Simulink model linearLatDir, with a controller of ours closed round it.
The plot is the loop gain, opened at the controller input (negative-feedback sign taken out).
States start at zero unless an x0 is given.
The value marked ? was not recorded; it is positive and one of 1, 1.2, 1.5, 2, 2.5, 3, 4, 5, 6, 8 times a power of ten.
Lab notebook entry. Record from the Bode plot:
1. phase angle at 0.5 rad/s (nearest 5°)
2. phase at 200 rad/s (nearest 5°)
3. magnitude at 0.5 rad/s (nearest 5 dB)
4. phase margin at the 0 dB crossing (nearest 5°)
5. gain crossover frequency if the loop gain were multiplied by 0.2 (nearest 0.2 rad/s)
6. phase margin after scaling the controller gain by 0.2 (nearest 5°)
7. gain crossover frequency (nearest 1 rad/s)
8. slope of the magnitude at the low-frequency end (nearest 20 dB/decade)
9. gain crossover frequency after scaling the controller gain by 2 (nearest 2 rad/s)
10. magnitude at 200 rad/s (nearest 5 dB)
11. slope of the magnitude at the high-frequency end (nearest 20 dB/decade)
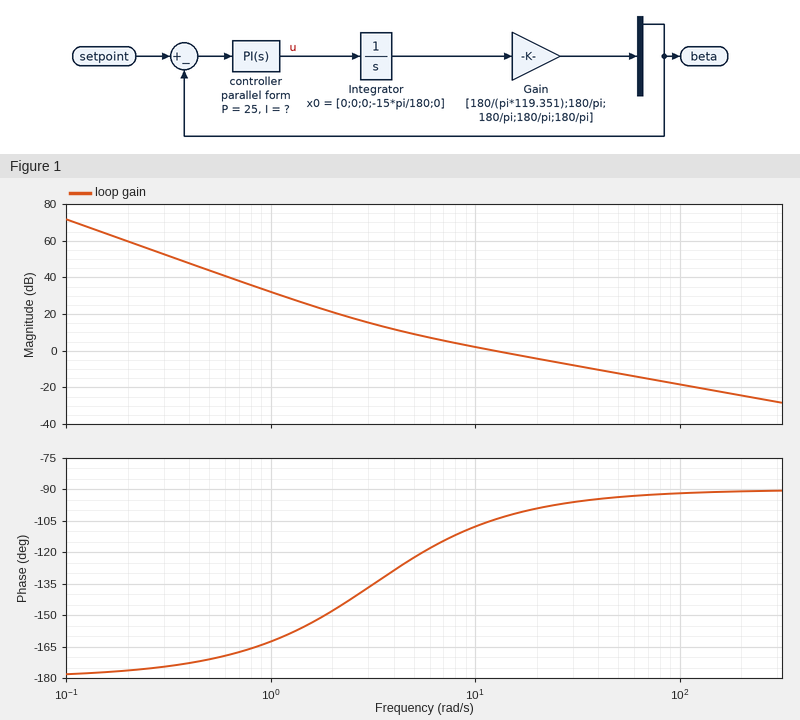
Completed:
-170°
-90°
45 dB
75°
3.4 rad/s
45°
12 rad/s
-40 dB/decade
24 rad/s
-25 dB
-20 dB/decade
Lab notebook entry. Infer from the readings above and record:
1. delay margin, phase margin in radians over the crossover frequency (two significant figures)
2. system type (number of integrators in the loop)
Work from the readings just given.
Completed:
0.11 s
2
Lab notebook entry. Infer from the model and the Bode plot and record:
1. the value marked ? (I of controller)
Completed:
80
